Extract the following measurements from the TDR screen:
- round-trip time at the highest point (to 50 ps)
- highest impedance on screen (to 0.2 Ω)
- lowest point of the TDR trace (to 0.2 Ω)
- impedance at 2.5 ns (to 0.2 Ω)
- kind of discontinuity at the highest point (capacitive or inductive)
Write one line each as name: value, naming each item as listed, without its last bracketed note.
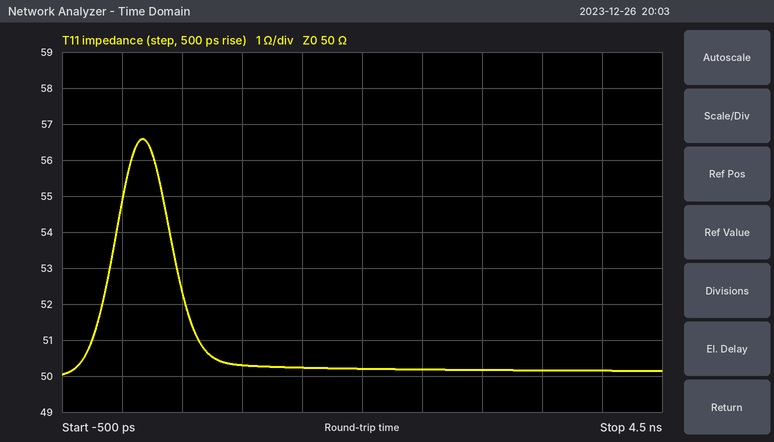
round-trip time at the highest point: 150 ps
highest impedance on screen: 56.6 Ω
lowest point of the TDR trace: 50.0 Ω
impedance at 2.5 ns: 50.2 Ω
kind of discontinuity at the highest point: inductive
